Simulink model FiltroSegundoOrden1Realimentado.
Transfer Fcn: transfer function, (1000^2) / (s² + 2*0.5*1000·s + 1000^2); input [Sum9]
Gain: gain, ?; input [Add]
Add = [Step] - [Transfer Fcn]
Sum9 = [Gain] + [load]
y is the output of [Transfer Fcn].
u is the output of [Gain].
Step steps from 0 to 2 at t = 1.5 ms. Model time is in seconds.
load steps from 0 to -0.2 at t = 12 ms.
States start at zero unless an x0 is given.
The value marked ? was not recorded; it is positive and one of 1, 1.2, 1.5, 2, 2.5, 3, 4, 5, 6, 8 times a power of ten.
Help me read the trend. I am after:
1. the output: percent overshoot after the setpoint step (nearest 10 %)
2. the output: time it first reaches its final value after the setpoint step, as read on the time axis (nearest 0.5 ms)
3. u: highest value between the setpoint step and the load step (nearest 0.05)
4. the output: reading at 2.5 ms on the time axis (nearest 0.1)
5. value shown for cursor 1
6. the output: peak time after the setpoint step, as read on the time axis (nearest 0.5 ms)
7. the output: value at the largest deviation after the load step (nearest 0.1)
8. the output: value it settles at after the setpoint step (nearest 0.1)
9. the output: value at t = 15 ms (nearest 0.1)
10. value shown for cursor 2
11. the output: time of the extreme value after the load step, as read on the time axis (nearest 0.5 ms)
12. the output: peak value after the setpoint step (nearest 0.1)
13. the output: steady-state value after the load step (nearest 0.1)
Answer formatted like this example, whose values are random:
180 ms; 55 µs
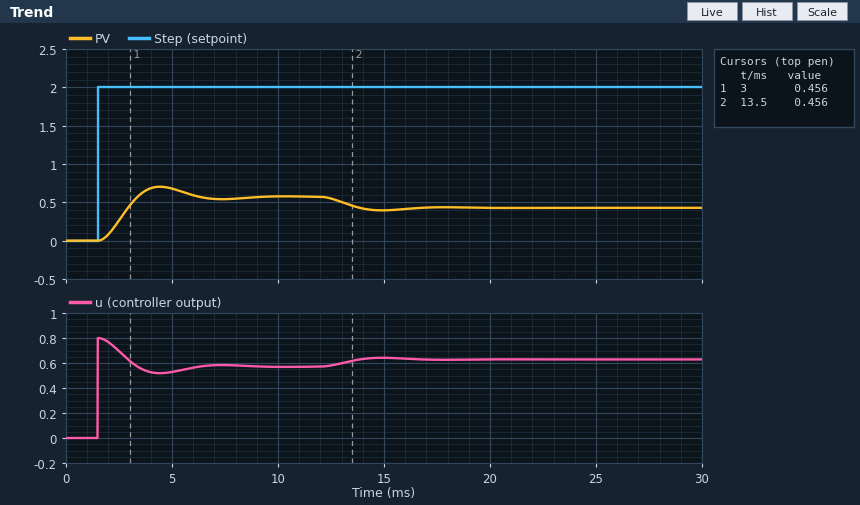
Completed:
20 %; 3.5 ms; 0.80; 0.3; 0.456; 4.5 ms; 0.4; 0.6; 0.4; 0.456; 15.0 ms; 0.7; 0.4
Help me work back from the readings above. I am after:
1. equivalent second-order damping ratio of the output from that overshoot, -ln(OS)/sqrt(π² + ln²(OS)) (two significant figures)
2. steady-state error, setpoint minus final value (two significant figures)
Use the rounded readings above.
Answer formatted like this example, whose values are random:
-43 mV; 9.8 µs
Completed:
0.46; 1.4
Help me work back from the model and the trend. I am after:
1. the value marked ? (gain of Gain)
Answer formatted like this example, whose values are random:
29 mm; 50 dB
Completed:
0.4
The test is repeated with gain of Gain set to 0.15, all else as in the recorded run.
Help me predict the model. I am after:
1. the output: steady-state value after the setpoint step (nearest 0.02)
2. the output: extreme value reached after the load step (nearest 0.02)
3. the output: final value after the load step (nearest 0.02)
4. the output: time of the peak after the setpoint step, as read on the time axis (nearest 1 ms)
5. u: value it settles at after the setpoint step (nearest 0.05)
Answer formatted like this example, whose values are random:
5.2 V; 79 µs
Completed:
0.26; 0.06; 0.08; 5 ms; 0.25
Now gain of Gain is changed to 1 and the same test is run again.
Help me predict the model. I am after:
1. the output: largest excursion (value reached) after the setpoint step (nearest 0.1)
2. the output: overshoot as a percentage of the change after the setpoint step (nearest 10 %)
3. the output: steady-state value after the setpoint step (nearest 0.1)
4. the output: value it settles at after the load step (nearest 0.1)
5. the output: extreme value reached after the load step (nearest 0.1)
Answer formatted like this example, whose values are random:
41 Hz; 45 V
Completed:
1.3; 30 %; 1.0; 0.9; 0.9
